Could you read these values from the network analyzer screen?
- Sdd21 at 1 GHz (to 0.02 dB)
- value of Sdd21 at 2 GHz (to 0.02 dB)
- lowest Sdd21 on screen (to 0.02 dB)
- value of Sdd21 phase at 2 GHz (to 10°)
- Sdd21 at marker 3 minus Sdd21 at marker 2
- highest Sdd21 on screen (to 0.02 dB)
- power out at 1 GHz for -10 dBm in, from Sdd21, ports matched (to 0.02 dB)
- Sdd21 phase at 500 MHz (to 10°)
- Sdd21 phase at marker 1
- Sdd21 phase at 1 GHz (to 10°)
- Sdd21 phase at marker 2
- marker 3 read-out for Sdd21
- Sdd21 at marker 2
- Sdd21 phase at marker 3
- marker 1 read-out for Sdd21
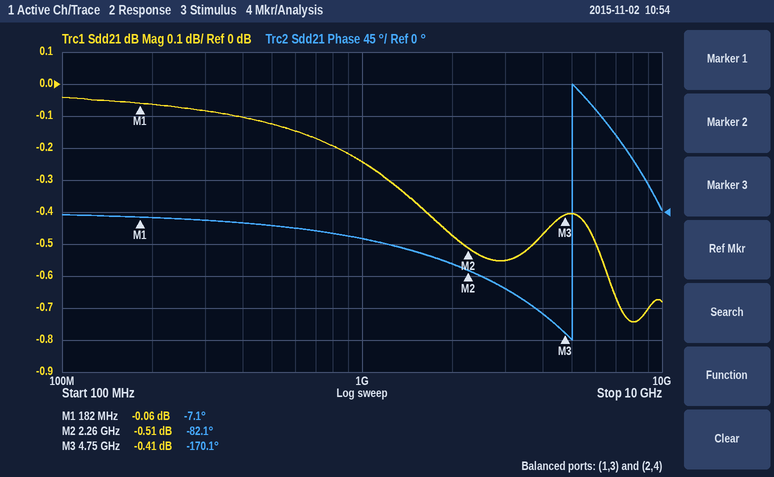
-0.24 dB
-0.48 dB
-0.74 dB
-70°
0.10 dB
-0.04 dB
-10.24 dBm
-20°
-7.1°
-40°
-82.1°
-0.41 dB
-0.51 dB
-170.1°
-0.06 dB
